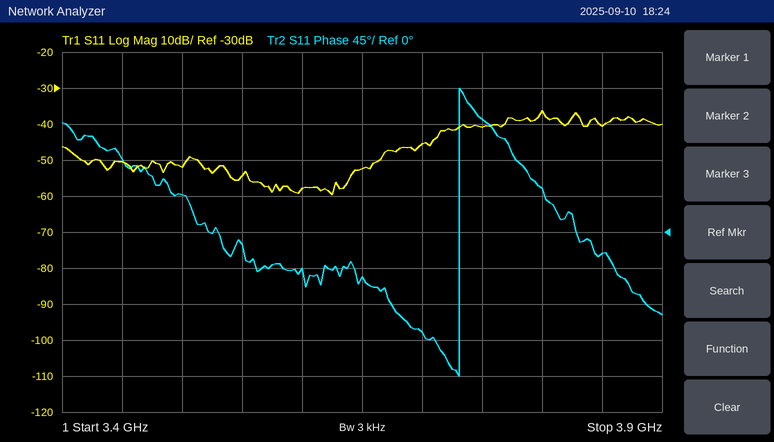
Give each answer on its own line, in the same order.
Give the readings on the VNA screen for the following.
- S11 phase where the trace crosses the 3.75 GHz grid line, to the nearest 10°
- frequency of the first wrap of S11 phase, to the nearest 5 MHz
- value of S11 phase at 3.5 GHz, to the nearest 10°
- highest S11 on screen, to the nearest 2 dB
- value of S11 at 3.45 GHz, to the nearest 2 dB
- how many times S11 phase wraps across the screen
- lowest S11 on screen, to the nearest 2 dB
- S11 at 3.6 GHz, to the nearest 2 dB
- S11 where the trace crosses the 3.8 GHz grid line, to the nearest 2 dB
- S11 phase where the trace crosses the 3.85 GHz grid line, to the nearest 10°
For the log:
140°
3.730 GHz
50°
-36 dB
-50 dB
1
-60 dB
-58 dB
-36 dB
-30°
